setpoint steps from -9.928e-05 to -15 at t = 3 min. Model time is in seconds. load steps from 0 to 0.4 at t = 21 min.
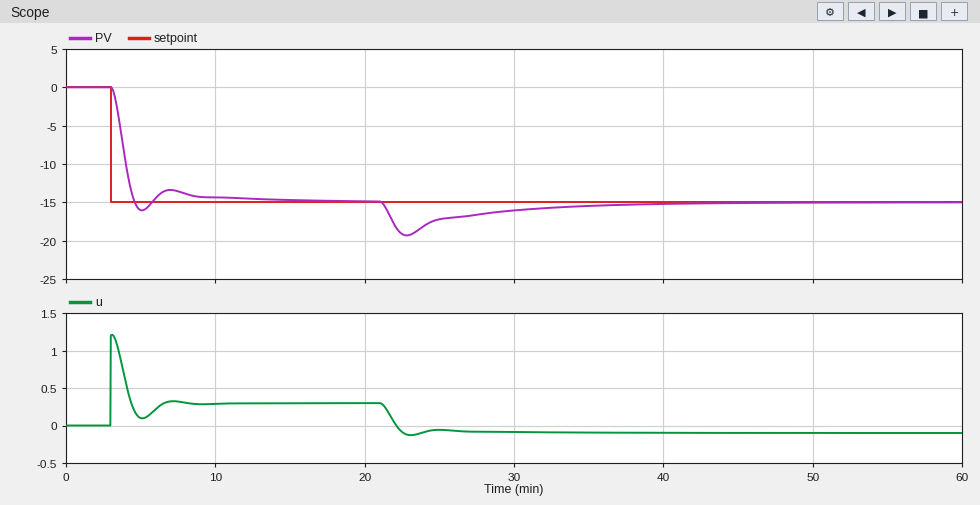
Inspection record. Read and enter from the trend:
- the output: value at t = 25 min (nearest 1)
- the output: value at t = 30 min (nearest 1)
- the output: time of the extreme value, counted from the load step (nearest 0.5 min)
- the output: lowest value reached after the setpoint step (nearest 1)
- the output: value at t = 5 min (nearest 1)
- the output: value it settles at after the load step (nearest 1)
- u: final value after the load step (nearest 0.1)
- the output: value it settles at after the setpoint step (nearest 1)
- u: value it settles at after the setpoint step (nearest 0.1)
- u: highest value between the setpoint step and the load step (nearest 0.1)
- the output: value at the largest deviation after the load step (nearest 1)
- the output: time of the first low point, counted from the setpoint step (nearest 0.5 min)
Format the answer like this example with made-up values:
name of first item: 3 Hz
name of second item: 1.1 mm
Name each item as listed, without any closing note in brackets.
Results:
the output: value at t = 25 min: -17
the output: value at t = 30 min: -16
the output: time of the extreme value, counted from the load step: 2.0 min
the output: lowest value reached after the setpoint step: -16
the output: value at t = 5 min: -16
the output: value it settles at after the load step: -15
u: final value after the load step: -0.1
the output: value it settles at after the setpoint step: -15
u: value it settles at after the setpoint step: 0.3
u: highest value between the setpoint step and the load step: 1.2
the output: value at the largest deviation after the load step: -19
the output: time of the first low point, counted from the setpoint step: 2.0 min
